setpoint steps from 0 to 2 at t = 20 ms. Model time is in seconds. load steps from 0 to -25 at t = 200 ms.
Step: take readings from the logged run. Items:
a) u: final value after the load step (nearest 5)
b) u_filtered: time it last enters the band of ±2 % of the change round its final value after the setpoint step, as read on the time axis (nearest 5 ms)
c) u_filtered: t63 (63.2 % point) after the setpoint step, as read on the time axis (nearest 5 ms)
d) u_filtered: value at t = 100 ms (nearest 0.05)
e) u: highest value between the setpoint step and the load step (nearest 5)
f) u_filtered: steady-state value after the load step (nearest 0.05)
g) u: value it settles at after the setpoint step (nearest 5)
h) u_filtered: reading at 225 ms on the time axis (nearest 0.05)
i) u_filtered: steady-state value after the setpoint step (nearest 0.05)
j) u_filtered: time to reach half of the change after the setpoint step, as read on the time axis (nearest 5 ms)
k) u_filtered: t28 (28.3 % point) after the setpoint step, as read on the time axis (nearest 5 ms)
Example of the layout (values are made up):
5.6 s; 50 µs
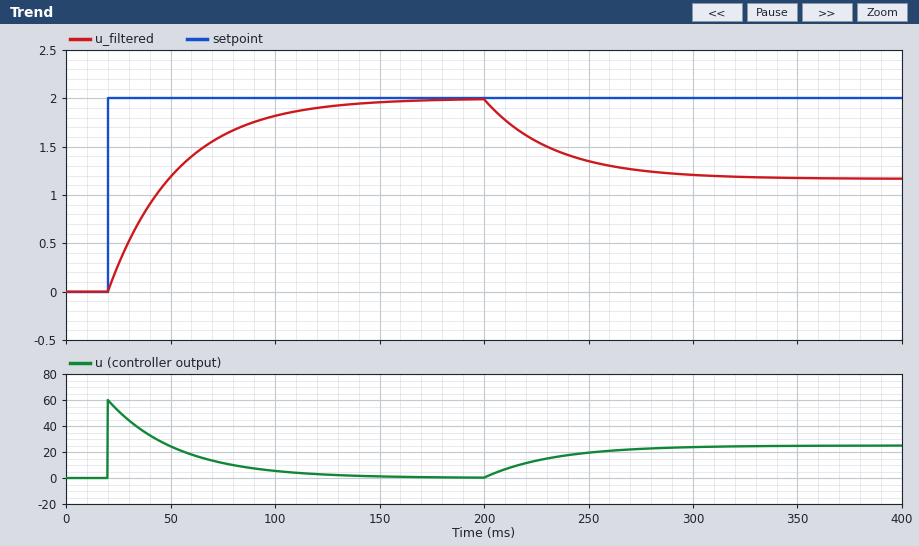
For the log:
25; 150 ms; 55 ms; 1.80; 60; 1.15; 0; 1.55; 2.00; 45 ms; 30 ms
